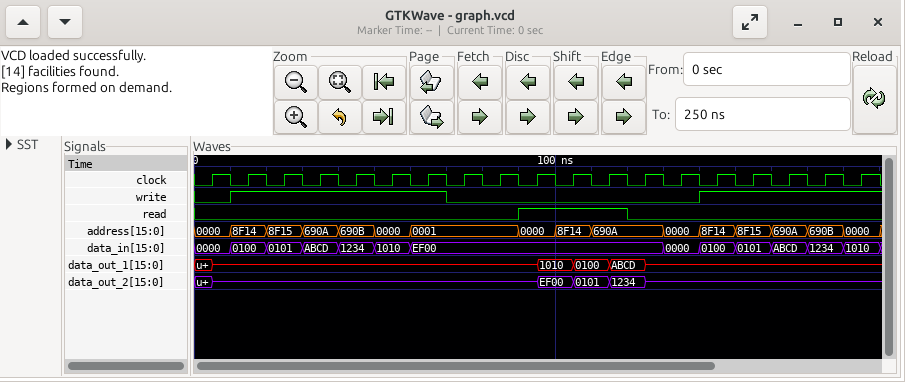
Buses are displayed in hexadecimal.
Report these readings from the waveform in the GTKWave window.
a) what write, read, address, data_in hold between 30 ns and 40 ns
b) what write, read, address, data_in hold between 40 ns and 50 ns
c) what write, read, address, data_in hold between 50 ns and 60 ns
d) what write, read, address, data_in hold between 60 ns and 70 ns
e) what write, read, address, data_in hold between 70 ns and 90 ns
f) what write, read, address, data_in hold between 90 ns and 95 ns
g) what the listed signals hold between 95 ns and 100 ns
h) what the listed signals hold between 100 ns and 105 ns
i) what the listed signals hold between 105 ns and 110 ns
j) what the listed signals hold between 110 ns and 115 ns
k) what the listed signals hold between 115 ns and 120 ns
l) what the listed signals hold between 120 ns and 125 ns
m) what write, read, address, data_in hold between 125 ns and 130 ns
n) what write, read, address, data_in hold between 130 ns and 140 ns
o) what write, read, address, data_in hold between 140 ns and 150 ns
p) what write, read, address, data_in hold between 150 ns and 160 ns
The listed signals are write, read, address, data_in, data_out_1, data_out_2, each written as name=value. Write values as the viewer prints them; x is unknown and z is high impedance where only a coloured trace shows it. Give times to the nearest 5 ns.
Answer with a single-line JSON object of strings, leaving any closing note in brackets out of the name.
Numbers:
{"what write, read, address, data_in hold between 30 ns and 40 ns": "write=1, read=0, address=690A, data_in=ABCD", "what write, read, address, data_in hold between 40 ns and 50 ns": "write=1, read=0, address=690B, data_in=1234", "what write, read, address, data_in hold between 50 ns and 60 ns": "write=1, read=0, address=0000, data_in=1010", "what write, read, address, data_in hold between 60 ns and 70 ns": "write=1, read=0, address=0001, data_in=EF00", "what write, read, address, data_in hold between 70 ns and 90 ns": "write=0, read=0, address=0001, data_in=EF00", "what write, read, address, data_in hold between 90 ns and 95 ns": "write=0, read=1, address=0000, data_in=EF00", "what the listed signals hold between 95 ns and 100 ns": "write=0, read=1, address=0000, data_in=EF00, data_out_1=1010, data_out_2=EF00", "what the listed signals hold between 100 ns and 105 ns": "write=0, read=1, address=8F14, data_in=EF00, data_out_1=1010, data_out_2=EF00", "what the listed signals hold between 105 ns and 110 ns": "write=0, read=1, address=8F14, data_in=EF00, data_out_1=0100, data_out_2=0101", "what the listed signals hold between 110 ns and 115 ns": "write=0, read=1, address=690A, data_in=EF00, data_out_1=0100, data_out_2=0101", "what the listed signals hold between 115 ns and 120 ns": "write=0, read=1, address=690A, data_in=EF00, data_out_1=ABCD, data_out_2=1234", "what the listed signals hold between 120 ns and 125 ns": "write=0, read=0, address=690A, data_in=EF00, data_out_1=ABCD, data_out_2=1234", "what write, read, address, data_in hold between 125 ns and 130 ns": "write=0, read=0, address=690A, data_in=EF00", "what write, read, address, data_in hold between 130 ns and 140 ns": "write=0, read=0, address=0000, data_in=0000", "what write, read, address, data_in hold between 140 ns and 150 ns": "write=1, read=0, address=8F14, data_in=0100", "what write, read, address, data_in hold between 150 ns and 160 ns": "write=1, read=0, address=8F15, data_in=0101"}
